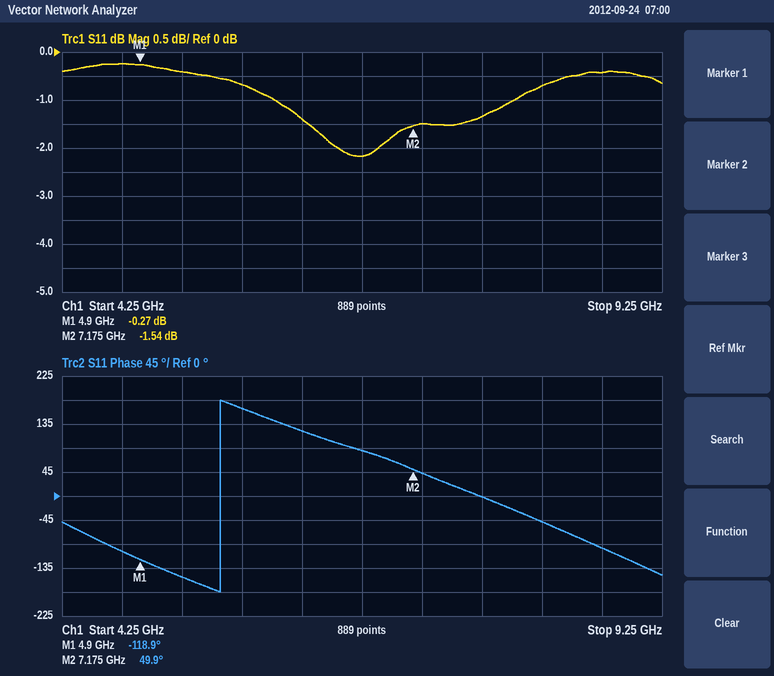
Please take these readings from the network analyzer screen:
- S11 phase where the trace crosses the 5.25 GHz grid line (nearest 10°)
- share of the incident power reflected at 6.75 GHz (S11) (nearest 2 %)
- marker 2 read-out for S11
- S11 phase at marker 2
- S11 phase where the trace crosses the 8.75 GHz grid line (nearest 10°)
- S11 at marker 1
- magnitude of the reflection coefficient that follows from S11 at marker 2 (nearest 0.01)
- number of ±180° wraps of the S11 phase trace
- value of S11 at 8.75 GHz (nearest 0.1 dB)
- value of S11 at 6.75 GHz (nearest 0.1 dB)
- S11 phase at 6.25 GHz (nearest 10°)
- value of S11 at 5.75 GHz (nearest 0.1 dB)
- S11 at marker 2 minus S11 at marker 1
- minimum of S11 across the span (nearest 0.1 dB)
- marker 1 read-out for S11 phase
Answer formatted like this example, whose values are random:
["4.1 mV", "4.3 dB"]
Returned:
["-150°", "60 %", "-1.54 dB", "49.9°", "-100°", "-0.27 dB", "0.84", "1", "-0.4 dB", "-2.2 dB", "120°", "-0.7 dB", "-1.27 dB", "-2.2 dB", "-118.9°"]
